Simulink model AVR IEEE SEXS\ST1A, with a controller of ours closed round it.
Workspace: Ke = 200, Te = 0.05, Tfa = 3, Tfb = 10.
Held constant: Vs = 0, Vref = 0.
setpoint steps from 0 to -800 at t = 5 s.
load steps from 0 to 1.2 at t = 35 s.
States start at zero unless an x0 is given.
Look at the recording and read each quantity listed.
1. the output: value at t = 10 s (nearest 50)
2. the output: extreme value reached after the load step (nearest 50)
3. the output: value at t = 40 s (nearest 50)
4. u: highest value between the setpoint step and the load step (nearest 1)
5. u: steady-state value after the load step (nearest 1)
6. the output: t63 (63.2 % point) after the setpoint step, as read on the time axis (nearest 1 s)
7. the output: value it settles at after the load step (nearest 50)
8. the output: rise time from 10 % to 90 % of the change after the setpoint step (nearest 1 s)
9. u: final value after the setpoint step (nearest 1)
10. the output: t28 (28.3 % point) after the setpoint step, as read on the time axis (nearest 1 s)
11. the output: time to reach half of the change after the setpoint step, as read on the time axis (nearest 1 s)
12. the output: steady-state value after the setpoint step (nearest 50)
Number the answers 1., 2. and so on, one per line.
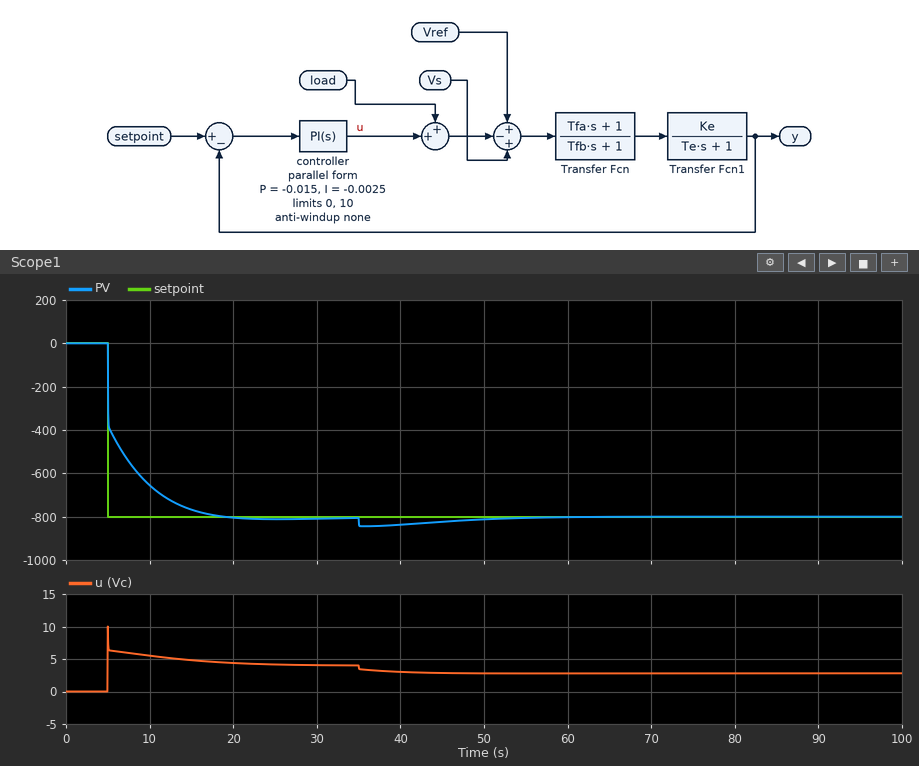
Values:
1. -650
2. -850
3. -850
4. 10
5. 3
6. 7 s
7. -800
8. 7 s
9. 4
10. 5 s
11. 5 s
12. -800
